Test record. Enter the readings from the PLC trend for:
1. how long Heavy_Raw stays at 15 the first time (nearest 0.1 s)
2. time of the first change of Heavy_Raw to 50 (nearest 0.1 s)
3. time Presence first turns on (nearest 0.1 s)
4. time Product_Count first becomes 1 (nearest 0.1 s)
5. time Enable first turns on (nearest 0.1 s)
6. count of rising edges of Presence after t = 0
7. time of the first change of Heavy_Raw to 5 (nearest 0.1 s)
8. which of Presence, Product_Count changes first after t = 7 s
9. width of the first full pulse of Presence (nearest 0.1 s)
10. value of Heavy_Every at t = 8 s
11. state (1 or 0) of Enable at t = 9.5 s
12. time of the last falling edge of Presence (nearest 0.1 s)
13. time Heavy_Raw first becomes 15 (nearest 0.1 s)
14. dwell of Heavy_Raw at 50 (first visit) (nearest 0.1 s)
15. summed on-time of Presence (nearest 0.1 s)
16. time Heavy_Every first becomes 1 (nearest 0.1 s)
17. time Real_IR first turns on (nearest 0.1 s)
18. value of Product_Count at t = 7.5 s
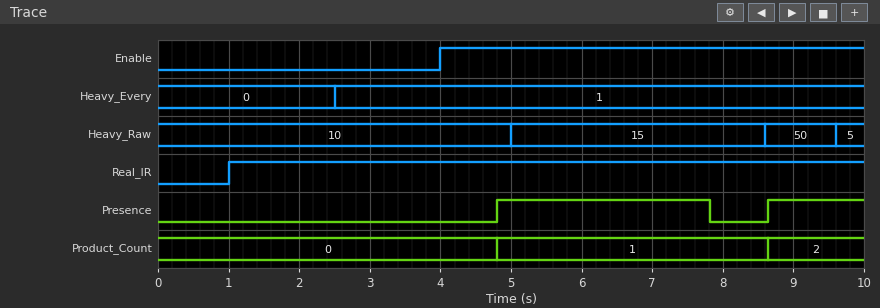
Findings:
3.6 s
8.6 s
4.8 s
4.8 s
4.0 s
2
9.6 s
Presence
3.0 s
1
1
7.8 s
5.0 s
1.0 s
4.4 s
2.5 s
1.0 s
1
